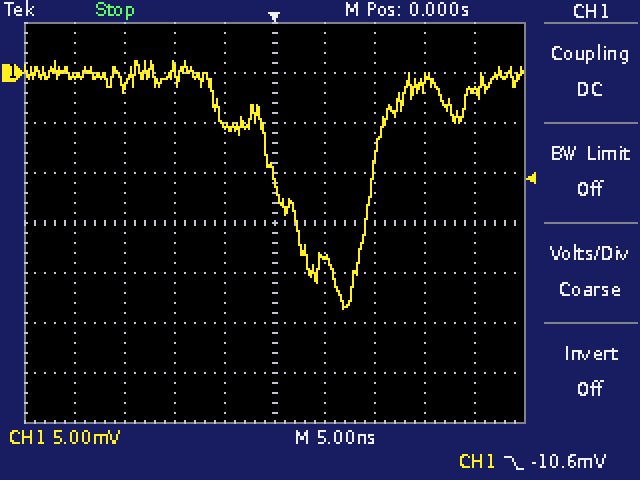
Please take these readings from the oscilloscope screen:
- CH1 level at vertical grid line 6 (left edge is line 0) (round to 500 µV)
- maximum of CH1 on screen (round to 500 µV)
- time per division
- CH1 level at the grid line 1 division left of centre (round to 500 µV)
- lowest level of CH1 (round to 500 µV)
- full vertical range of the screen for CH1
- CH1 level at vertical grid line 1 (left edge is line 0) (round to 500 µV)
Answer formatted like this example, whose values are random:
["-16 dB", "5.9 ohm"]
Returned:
["-18.5 mV", "1.0 mV", "5 ns", "-5.0 mV", "-23.5 mV", "40 mV", "-500 µV"]
